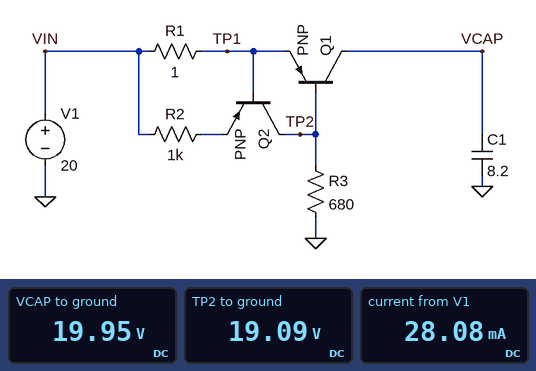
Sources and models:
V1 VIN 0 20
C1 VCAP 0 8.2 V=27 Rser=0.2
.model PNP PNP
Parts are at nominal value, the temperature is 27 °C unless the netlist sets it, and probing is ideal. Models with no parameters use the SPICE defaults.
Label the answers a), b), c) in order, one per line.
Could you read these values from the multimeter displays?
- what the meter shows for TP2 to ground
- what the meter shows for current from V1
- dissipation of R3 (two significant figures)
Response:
a) 19.09 V
b) 28.08 mA
c) 540 mW
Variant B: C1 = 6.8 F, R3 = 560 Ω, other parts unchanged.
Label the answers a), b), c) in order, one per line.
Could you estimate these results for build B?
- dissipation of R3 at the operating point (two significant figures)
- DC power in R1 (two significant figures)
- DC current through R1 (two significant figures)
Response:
a) 650 mW
b) 1.2 mW
c) 34 mA
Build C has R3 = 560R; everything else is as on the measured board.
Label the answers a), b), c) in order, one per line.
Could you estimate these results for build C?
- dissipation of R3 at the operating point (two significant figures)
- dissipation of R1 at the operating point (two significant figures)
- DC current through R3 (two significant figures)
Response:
a) 650 mW
b) 1.2 mW
c) 34 mA
